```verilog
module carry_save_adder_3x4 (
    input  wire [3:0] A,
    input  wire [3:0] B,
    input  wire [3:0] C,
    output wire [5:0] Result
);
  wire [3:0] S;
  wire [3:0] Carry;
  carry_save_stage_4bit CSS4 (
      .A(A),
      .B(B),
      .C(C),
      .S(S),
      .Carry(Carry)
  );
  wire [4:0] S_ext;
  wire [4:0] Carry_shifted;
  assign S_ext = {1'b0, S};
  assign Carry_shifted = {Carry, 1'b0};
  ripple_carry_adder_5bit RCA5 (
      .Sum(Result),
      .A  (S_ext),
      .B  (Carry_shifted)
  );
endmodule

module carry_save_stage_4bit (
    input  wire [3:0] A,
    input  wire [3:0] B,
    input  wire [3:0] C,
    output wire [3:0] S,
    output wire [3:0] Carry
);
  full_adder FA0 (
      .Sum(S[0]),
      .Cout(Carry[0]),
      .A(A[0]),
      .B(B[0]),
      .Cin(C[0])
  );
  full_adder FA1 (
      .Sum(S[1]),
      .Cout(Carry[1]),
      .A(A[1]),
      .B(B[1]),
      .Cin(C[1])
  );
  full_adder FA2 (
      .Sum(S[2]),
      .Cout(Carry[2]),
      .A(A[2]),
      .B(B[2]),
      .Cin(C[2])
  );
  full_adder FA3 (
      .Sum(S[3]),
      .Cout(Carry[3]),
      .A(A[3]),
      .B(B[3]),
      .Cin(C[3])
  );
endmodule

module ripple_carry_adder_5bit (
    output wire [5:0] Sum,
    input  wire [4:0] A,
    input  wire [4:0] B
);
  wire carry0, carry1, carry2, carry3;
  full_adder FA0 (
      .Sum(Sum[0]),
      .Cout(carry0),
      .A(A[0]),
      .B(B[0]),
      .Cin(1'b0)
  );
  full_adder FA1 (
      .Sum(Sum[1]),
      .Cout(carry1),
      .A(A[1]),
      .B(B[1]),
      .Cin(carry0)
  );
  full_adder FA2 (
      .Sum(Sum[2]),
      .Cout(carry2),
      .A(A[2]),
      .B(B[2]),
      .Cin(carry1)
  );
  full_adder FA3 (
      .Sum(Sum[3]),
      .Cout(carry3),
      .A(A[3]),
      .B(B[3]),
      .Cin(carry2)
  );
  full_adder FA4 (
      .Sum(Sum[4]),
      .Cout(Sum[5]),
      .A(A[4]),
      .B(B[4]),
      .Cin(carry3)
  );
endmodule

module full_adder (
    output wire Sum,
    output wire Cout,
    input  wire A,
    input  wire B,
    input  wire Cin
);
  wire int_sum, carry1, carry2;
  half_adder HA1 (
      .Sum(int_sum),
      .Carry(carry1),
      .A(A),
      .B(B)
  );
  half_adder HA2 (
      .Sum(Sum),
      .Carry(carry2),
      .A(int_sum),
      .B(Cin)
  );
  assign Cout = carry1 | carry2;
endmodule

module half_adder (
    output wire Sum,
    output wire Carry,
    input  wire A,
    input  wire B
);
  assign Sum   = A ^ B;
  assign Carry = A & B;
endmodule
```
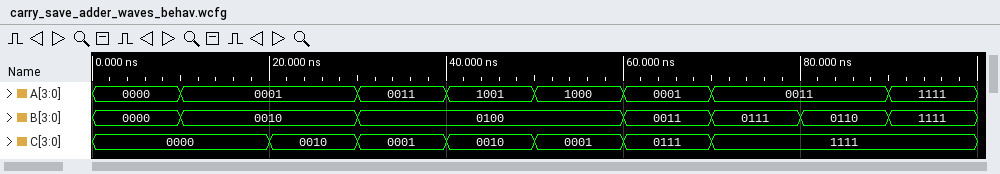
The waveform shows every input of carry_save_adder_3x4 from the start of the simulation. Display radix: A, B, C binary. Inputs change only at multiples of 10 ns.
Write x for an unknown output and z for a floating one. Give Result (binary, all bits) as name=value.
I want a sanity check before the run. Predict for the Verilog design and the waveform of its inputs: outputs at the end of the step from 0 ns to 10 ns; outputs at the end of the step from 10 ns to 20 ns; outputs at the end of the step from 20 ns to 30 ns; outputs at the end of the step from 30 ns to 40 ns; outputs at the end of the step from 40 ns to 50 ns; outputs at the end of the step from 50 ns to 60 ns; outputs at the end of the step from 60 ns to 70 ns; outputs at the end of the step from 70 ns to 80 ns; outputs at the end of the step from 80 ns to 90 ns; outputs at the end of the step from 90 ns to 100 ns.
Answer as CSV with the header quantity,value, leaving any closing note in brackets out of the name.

quantity,value
outputs at the end of the step from 0 ns to 10 ns,Result=000000
outputs at the end of the step from 10 ns to 20 ns,Result=000011
outputs at the end of the step from 20 ns to 30 ns,Result=000101
outputs at the end of the step from 30 ns to 40 ns,Result=001000
outputs at the end of the step from 40 ns to 50 ns,Result=001111
outputs at the end of the step from 50 ns to 60 ns,Result=001101
outputs at the end of the step from 60 ns to 70 ns,Result=001011
outputs at the end of the step from 70 ns to 80 ns,Result=011001
outputs at the end of the step from 80 ns to 90 ns,Result=011000
outputs at the end of the step from 90 ns to 100 ns,Result=101101
